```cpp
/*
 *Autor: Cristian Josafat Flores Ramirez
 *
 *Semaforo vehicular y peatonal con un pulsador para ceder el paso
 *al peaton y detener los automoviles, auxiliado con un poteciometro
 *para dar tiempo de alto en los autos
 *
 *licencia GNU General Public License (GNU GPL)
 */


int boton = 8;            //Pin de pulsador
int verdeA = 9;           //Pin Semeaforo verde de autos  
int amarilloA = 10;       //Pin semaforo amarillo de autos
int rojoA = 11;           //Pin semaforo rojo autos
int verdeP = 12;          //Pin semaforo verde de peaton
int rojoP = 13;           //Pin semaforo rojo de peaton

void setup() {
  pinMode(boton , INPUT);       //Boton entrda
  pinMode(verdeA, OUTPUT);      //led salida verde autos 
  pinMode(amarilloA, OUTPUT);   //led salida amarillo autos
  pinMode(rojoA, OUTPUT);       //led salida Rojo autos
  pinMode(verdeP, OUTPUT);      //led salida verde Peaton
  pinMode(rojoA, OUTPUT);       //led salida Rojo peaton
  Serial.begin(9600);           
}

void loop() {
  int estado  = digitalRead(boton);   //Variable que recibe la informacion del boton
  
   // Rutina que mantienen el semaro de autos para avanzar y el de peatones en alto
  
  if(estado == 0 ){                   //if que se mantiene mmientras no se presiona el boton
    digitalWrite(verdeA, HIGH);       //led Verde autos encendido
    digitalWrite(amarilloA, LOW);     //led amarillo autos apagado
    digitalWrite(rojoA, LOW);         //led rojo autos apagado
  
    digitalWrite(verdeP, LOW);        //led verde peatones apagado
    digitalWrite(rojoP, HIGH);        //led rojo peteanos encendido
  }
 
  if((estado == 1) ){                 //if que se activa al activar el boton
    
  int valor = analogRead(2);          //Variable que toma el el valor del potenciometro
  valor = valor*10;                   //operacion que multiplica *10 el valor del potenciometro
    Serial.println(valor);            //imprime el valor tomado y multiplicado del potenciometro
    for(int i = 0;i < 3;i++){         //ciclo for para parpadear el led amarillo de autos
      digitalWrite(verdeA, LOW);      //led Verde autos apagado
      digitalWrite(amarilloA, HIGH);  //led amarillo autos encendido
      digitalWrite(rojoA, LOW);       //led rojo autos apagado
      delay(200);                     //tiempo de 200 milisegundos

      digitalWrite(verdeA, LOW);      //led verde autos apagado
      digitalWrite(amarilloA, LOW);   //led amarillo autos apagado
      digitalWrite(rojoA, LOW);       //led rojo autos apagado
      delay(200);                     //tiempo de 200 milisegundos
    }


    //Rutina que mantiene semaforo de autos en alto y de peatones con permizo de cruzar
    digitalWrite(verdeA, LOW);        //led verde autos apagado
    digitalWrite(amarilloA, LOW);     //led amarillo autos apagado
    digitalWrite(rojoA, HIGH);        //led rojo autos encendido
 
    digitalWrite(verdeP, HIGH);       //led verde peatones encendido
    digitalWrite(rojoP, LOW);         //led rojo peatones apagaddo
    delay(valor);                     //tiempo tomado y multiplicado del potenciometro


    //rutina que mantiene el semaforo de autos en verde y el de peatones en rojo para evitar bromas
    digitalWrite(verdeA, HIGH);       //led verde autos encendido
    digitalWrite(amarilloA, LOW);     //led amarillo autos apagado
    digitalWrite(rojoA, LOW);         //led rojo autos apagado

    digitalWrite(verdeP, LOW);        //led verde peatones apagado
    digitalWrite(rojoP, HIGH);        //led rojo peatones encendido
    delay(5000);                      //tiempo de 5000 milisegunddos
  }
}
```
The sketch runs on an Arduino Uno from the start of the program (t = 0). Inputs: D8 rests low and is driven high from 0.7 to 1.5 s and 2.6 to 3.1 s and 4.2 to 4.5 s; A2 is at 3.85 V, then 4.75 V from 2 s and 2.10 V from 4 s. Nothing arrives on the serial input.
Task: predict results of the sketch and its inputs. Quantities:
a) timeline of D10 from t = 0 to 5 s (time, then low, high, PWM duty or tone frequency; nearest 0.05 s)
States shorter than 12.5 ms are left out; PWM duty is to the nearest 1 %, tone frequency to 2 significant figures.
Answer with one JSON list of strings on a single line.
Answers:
["0 s low; 0.7 s high; 0.9 s low; 1.1 s high; 1.3 s low; 1.5 s high; 1.7 s low"]
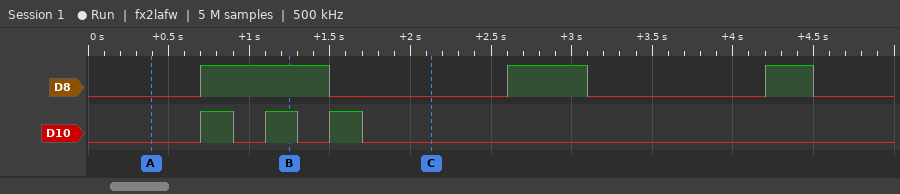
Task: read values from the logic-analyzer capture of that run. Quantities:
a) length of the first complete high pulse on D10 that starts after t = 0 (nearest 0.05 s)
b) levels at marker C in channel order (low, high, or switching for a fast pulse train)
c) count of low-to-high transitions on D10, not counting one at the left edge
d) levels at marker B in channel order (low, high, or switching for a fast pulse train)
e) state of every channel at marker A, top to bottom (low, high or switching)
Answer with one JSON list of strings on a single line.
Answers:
["0.20 s", "D8 low, D10 low", "3", "D8 high, D10 high", "D8 low, D10 low"]
